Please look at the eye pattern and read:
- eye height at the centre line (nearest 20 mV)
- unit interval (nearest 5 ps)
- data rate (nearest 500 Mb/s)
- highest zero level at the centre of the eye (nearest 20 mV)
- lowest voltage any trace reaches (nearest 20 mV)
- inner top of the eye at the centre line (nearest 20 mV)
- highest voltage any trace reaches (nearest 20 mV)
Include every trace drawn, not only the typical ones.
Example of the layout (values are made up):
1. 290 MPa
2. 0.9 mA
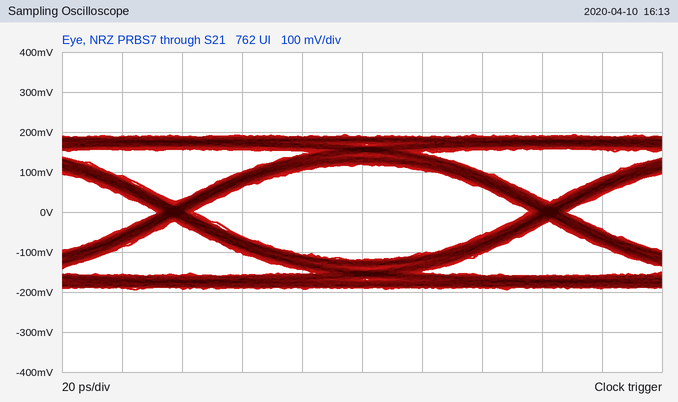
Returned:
1. 240 mV
2. 125 ps
3. 8.0 Gb/s
4. -120 mV
5. -200 mV
6. 120 mV
7. 200 mV
